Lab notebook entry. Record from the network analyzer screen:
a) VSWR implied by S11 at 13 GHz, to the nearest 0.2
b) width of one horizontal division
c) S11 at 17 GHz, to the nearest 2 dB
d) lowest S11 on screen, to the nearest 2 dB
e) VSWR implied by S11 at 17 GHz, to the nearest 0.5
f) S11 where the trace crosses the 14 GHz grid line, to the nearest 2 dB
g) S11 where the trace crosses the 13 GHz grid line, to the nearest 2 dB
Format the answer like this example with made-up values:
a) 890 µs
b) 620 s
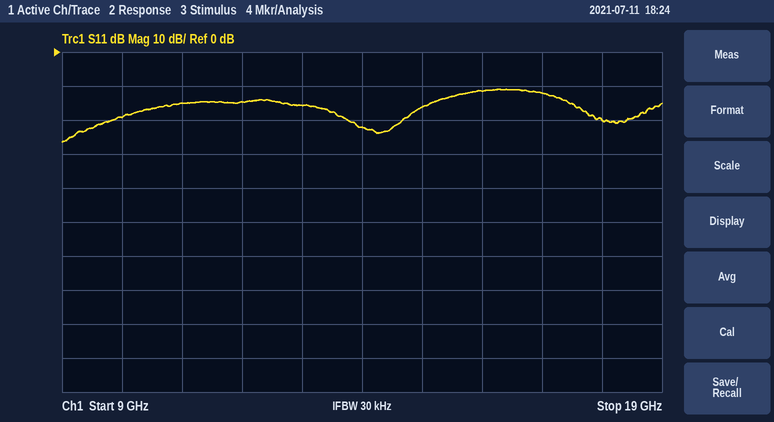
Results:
a) 1.4
b) 1 GHz
c) -12 dB
d) -26 dB
e) 1.5
f) -22 dB
g) -16 dB
